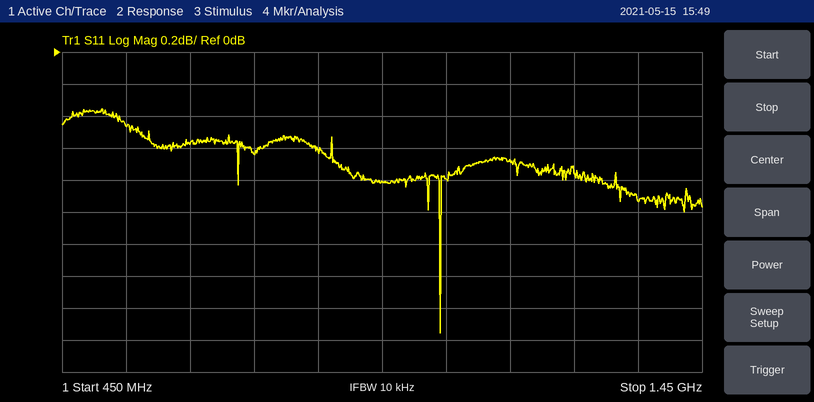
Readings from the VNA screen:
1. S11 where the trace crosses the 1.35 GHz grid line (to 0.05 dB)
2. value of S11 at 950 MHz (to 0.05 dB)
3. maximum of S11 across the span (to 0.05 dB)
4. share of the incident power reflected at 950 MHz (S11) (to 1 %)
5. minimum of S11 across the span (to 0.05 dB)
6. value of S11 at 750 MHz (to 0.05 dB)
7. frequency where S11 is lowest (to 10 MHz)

-0.95 dB
-0.80 dB
-0.35 dB
83 %
-1.75 dB
-0.65 dB
1.04 GHz
